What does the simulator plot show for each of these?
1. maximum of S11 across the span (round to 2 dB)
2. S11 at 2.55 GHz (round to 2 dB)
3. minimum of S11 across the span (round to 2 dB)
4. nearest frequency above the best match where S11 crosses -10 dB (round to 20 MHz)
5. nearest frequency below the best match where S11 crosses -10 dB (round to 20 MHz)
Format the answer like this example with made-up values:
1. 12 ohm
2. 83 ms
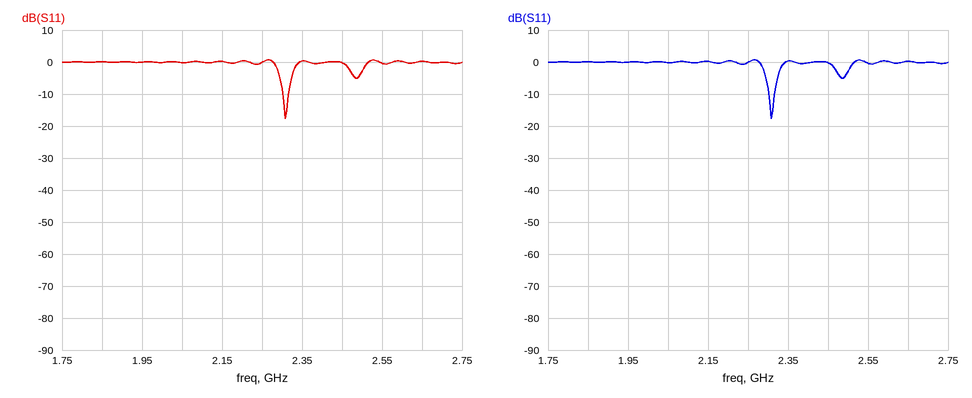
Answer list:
1. 0 dB
2. 0 dB
3. -18 dB
4. 2.32 GHz
5. 2.30 GHz
